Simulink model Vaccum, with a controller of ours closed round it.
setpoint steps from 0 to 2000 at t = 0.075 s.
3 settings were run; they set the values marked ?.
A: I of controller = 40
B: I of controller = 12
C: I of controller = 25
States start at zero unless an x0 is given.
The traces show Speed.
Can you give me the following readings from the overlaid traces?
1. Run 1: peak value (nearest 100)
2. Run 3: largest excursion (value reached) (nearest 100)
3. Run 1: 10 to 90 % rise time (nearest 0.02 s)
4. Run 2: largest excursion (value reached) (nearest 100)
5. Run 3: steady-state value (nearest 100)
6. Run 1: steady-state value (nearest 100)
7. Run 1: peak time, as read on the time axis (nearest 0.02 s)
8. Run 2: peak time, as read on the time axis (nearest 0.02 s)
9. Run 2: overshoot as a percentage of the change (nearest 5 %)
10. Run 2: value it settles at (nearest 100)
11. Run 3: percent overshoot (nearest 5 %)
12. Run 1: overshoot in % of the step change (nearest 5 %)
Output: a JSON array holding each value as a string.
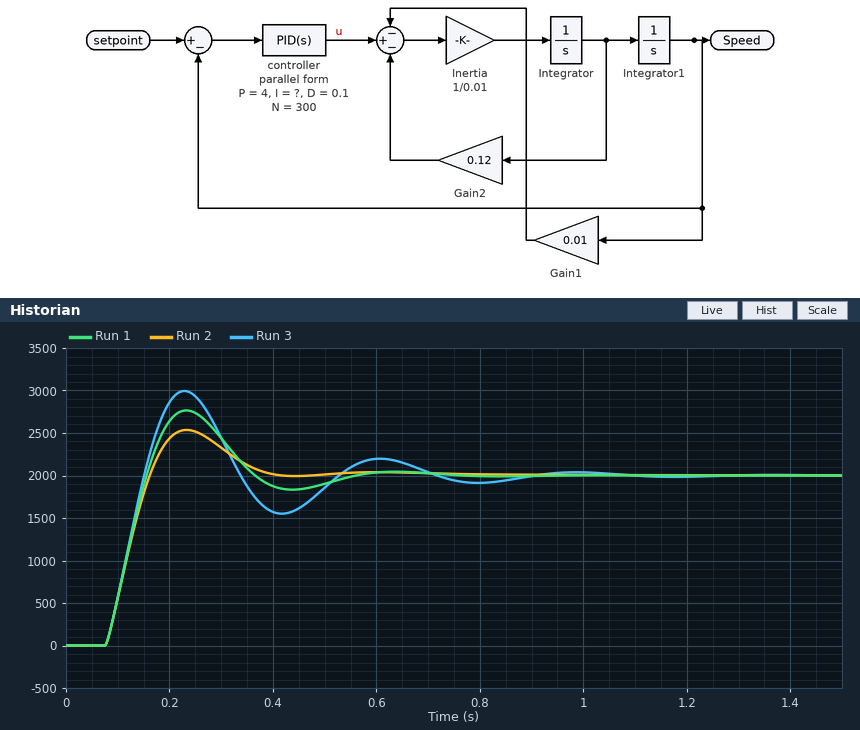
["2800", "3000", "0.06 s", "2500", "2000", "2000", "0.24 s", "0.24 s", "25 %", "2000", "50 %", "40 %"]
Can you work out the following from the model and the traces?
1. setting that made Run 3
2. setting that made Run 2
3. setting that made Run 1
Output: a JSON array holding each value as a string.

["A", "B", "C"]
